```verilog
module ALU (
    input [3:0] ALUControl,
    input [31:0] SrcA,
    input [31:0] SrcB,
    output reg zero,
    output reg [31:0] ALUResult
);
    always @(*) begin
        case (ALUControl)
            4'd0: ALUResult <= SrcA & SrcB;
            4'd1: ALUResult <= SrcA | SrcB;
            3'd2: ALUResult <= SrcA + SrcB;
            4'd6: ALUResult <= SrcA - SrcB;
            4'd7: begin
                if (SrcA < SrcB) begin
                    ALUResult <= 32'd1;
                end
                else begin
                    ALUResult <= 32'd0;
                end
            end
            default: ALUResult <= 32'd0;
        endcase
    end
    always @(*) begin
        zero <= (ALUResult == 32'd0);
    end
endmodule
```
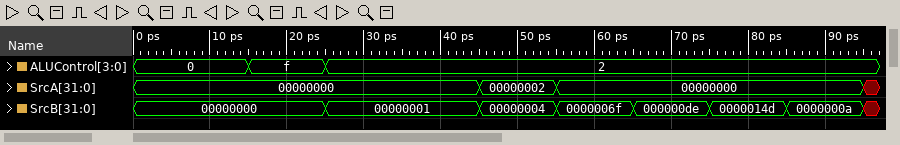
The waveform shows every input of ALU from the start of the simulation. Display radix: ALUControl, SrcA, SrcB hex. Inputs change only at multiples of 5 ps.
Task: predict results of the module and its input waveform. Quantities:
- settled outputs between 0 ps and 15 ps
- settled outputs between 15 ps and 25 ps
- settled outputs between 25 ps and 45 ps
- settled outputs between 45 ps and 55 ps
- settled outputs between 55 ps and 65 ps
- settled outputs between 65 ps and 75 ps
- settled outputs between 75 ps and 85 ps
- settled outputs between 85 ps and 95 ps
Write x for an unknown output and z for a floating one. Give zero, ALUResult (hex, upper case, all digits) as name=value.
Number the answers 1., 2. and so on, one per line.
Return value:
1. zero=1, ALUResult=00000000
2. zero=1, ALUResult=00000000
3. zero=0, ALUResult=00000001
4. zero=0, ALUResult=00000006
5. zero=0, ALUResult=0000006F
6. zero=0, ALUResult=000000DE
7. zero=0, ALUResult=0000014D
8. zero=0, ALUResult=0000000A
